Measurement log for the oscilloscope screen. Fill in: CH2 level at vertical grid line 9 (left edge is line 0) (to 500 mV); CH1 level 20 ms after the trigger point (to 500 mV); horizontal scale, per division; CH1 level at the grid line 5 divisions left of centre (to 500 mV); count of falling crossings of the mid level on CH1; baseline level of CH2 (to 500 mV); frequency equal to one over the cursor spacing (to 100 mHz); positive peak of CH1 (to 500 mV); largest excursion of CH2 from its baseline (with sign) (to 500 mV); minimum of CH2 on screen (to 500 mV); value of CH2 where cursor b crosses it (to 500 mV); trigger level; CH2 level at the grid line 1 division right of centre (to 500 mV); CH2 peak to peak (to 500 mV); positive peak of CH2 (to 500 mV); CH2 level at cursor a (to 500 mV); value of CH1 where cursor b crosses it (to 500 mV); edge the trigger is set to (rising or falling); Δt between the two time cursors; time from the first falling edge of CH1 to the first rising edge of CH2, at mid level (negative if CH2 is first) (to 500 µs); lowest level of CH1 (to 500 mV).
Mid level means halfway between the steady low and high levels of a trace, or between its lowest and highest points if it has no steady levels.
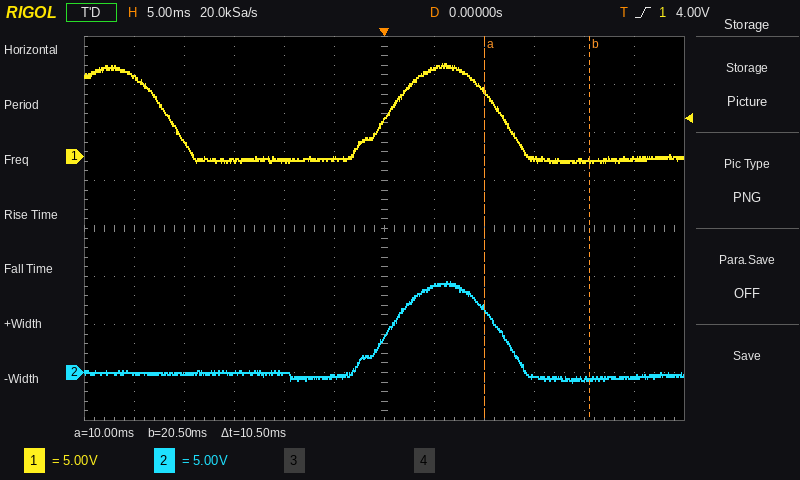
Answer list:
-500 mV
-500 mV
5 ms
8.5 V
2
0.0 V
95.2 Hz
9.5 V
+9.5 V
-1.0 V
-500 mV
4.00 V
9.0 V
10.5 V
9.5 V
6.5 V
-500 mV
rising
10.5 ms
+22.0 ms
-500 mV
